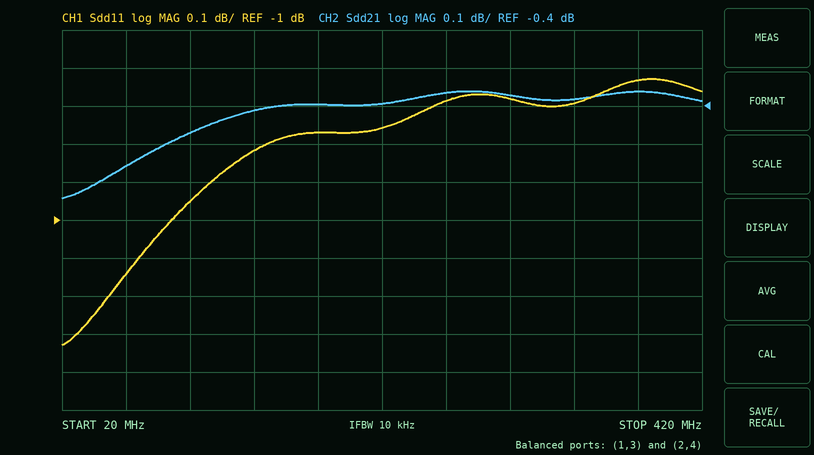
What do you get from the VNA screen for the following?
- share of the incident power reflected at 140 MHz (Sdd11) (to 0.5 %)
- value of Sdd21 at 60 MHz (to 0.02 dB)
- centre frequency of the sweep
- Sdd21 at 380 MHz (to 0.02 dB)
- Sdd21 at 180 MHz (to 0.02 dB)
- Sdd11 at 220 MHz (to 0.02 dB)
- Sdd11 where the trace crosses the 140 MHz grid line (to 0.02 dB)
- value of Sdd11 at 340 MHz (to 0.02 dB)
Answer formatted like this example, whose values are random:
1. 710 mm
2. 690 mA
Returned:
1. 83.0 %
2. -0.56 dB
3. 220 MHz
4. -0.36 dB
5. -0.40 dB
6. -0.76 dB
7. -0.82 dB
8. -0.70 dB
